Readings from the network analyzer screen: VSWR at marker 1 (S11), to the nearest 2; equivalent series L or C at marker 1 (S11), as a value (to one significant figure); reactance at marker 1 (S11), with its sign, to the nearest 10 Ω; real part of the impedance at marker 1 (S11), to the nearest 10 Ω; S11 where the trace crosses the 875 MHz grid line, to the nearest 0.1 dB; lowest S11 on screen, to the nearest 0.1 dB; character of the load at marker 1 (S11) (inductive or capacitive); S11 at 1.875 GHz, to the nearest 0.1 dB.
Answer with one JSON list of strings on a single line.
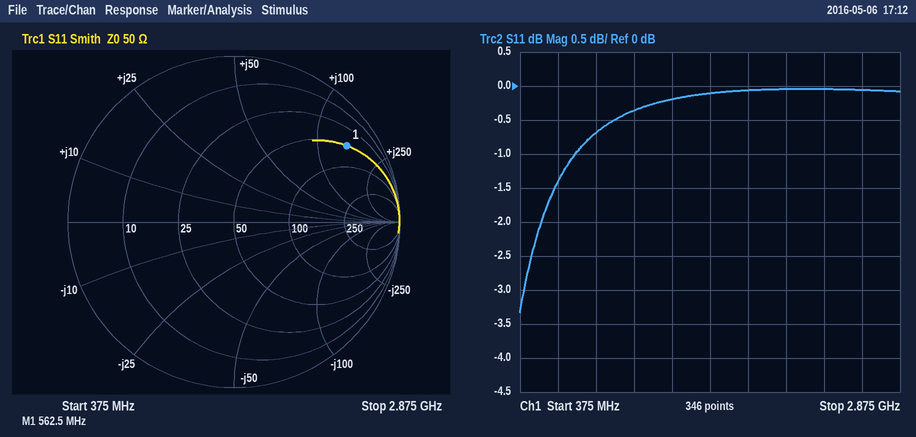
["10", "40 nH", "+150 Ω", "50 Ω", "-0.7 dB", "-3.3 dB", "inductive", "-0.1 dB"]
